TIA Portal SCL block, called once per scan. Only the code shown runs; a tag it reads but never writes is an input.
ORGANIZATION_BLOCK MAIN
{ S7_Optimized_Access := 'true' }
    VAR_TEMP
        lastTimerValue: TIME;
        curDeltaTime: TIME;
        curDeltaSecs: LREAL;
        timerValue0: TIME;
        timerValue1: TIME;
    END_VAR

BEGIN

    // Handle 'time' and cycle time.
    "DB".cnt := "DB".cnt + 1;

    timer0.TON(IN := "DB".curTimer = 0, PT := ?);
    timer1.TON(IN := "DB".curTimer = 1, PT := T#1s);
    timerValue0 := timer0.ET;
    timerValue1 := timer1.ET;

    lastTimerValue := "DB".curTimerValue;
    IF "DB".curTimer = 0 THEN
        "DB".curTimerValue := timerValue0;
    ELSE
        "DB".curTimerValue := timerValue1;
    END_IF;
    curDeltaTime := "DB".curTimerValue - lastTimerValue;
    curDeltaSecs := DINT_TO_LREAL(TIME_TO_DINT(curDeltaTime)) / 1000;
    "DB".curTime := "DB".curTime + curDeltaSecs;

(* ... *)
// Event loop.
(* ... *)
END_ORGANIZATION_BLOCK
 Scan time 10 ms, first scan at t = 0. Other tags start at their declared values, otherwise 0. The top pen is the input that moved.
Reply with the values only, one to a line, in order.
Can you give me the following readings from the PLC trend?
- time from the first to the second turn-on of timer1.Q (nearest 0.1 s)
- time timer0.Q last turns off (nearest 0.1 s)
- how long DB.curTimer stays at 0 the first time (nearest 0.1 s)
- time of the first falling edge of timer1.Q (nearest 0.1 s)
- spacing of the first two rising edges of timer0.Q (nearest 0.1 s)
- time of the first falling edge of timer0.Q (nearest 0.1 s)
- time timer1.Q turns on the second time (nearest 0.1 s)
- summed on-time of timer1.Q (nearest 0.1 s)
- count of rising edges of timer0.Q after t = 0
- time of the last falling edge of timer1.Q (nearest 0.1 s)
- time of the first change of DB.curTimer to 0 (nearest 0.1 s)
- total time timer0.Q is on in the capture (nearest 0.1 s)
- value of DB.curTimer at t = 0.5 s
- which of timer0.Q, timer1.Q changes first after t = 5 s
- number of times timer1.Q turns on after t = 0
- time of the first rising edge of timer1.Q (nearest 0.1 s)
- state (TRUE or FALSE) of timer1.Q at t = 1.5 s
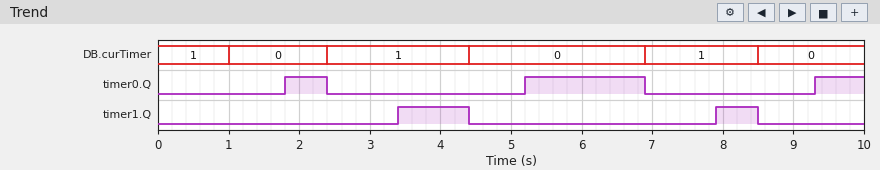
4.5 s
6.9 s
1.4 s
4.4 s
3.4 s
2.4 s
7.9 s
1.6 s
3
8.5 s
1.0 s
3.0 s
1
timer0.Q
2
3.4 s
FALSE
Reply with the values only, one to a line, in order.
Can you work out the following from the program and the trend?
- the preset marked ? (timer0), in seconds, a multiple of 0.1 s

0.8 s
